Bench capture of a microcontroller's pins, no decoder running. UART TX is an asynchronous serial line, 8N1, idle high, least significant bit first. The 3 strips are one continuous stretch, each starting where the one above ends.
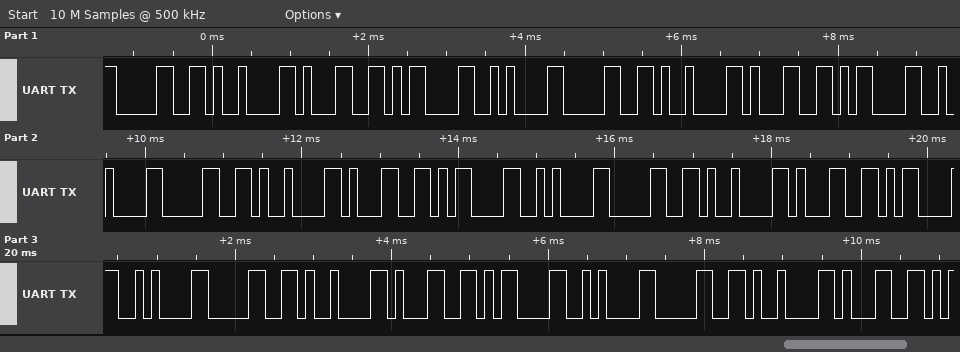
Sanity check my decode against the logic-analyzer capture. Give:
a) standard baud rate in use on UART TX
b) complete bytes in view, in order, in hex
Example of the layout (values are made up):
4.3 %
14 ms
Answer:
9600 baud
30 09 31 0D 0A 30 09 31 0D 0A 30 09 31 0D 0A 30 09 31 0D 0A 30 09 31 0D 0A 30 09 31
